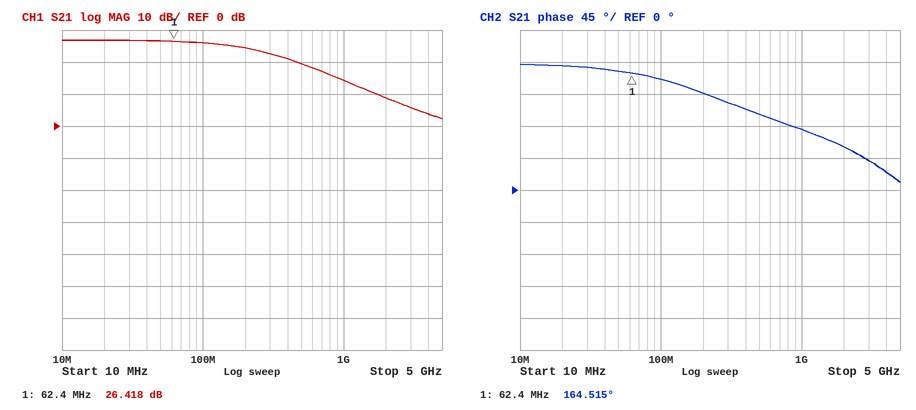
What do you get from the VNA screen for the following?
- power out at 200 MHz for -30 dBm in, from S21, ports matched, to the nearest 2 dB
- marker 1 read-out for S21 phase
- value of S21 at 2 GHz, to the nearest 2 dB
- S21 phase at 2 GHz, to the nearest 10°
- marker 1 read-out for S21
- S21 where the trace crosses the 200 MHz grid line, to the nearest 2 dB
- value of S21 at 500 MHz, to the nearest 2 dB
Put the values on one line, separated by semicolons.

-6 dBm; 164.515°; 8 dB; 60°; 26.418 dB; 24 dB; 20 dB
